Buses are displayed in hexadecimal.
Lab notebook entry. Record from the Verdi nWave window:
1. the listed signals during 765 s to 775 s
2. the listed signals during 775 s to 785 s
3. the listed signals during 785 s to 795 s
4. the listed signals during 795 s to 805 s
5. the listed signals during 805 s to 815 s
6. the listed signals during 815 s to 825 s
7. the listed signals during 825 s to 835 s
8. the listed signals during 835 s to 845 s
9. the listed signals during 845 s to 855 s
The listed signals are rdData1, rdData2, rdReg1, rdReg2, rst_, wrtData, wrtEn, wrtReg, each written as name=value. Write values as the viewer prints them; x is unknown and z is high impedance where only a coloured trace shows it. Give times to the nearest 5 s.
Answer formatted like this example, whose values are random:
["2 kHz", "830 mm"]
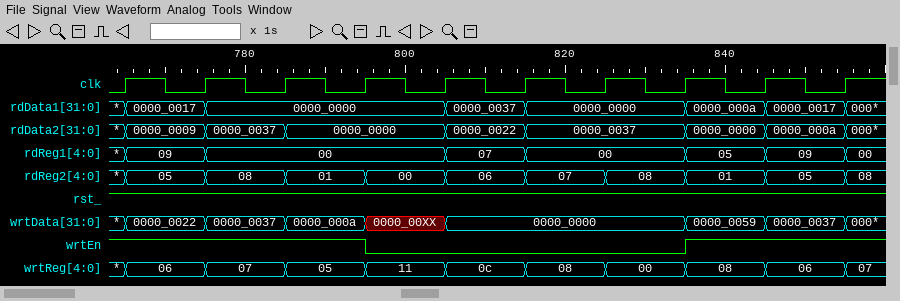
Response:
["rdData1=0000_0017, rdData2=0000_0009, rdReg1=09, rdReg2=05, rst_=1, wrtData=0000_0022, wrtEn=1, wrtReg=06", "rdData1=0000_0000, rdData2=0000_0037, rdReg1=00, rdReg2=08, rst_=1, wrtData=0000_0037, wrtEn=1, wrtReg=07", "rdData1=0000_0000, rdData2=0000_0000, rdReg1=00, rdReg2=01, rst_=1, wrtData=0000_000a, wrtEn=1, wrtReg=05", "rdData1=0000_0000, rdData2=0000_0000, rdReg1=00, rdReg2=00, rst_=1, wrtData=0000_00XX, wrtEn=0, wrtReg=11", "rdData1=0000_0037, rdData2=0000_0022, rdReg1=07, rdReg2=06, rst_=1, wrtData=0000_0000, wrtEn=0, wrtReg=0c", "rdData1=0000_0000, rdData2=0000_0037, rdReg1=00, rdReg2=07, rst_=1, wrtData=0000_0000, wrtEn=0, wrtReg=08", "rdData1=0000_0000, rdData2=0000_0037, rdReg1=00, rdReg2=08, rst_=1, wrtData=0000_0000, wrtEn=0, wrtReg=00", "rdData1=0000_000a, rdData2=0000_0000, rdReg1=05, rdReg2=01, rst_=1, wrtData=0000_0059, wrtEn=1, wrtReg=08", "rdData1=0000_0017, rdData2=0000_000a, rdReg1=09, rdReg2=05, rst_=1, wrtData=0000_0037, wrtEn=1, wrtReg=06"]
